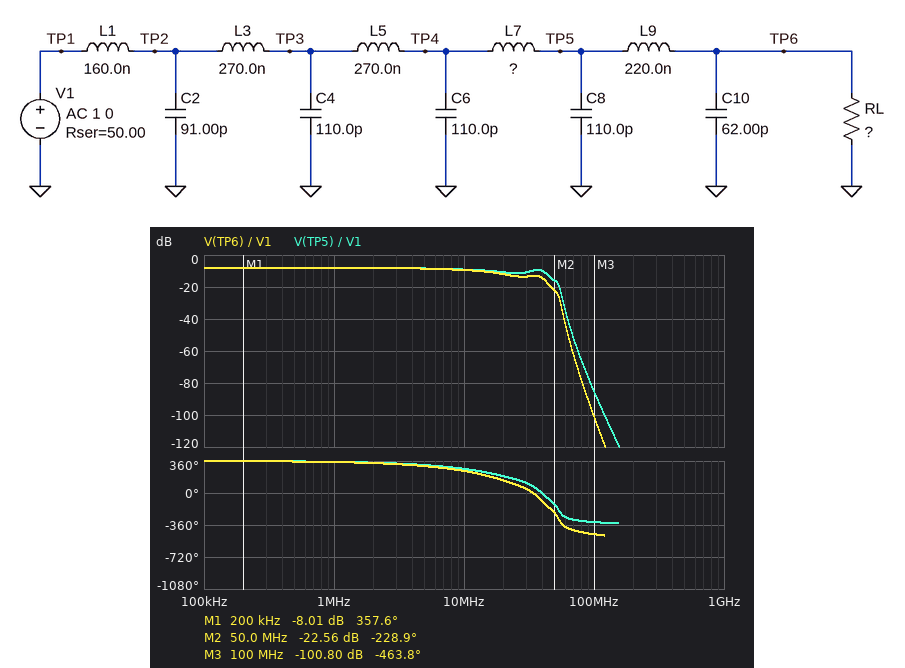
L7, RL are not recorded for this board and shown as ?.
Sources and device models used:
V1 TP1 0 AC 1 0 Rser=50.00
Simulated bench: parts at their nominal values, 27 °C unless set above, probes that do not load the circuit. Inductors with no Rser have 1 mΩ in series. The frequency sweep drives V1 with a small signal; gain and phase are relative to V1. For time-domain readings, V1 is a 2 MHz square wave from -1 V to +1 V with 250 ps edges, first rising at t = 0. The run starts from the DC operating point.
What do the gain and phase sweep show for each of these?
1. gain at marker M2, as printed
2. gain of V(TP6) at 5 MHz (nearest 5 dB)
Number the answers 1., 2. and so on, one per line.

1. -22.56 dB
2. -10 dB
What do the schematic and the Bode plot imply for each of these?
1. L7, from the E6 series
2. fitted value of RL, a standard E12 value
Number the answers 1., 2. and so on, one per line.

1. 1 µH
2. 33 Ω
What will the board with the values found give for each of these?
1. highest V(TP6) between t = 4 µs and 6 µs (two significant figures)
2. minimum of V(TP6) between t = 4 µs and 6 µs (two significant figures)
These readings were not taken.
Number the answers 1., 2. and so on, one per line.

1. 410 mV
2. -410 mV
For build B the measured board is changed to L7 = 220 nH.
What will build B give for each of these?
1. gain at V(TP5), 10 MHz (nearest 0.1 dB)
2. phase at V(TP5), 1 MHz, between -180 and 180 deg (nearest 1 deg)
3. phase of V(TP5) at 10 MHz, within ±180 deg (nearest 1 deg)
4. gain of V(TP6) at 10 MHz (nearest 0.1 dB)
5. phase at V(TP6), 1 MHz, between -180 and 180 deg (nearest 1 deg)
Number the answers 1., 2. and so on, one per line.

1. -7.7 dB
2. -6 deg
3. -60 deg
4. -8.0 dB
5. -8 deg
